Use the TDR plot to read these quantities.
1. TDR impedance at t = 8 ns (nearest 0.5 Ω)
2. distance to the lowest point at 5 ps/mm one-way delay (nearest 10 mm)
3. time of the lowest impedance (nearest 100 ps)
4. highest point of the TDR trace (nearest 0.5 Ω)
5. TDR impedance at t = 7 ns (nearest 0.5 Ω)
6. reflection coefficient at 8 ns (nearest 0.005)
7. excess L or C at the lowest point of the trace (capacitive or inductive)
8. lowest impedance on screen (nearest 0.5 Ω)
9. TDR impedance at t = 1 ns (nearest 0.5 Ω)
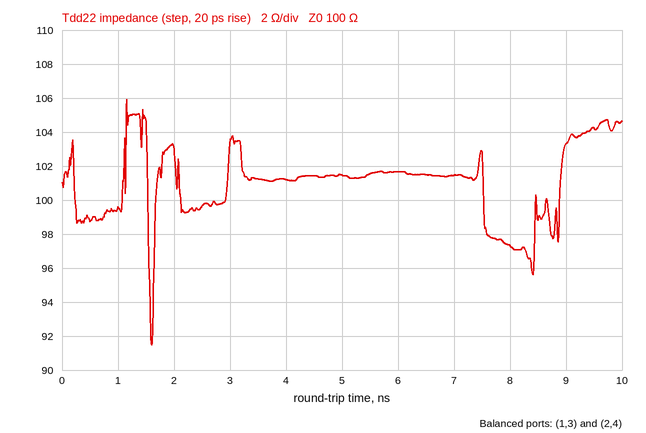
97.5 Ω
160 mm
1.6 ns
106.0 Ω
101.5 Ω
-0.015
capacitive
91.5 Ω
99.5 Ω
